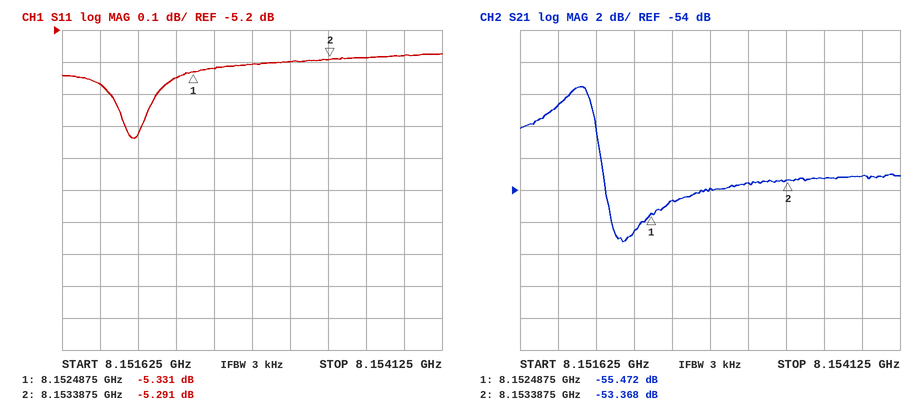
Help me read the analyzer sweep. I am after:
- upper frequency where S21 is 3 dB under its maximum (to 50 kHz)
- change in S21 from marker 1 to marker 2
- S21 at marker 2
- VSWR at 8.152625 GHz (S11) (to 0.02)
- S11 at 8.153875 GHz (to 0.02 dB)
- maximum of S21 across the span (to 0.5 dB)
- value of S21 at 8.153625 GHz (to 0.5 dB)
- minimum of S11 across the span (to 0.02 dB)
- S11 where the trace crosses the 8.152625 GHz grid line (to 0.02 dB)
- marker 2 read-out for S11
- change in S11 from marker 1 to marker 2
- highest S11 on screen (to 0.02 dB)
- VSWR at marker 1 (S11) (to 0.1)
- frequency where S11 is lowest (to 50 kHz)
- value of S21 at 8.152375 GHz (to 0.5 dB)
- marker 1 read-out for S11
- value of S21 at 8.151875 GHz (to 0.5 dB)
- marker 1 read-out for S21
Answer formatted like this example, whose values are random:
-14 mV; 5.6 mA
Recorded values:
8.15215 GHz; 2.104 dB; -53.368 dB; 3.36; -5.28 dB; -47.5 dB; -53.5 dB; -5.54 dB; -5.32 dB; -5.291 dB; 0.040 dB; -5.28 dB; 3.4; 8.15210 GHz; -56.5 dB; -5.331 dB; -48.5 dB; -55.472 dB
